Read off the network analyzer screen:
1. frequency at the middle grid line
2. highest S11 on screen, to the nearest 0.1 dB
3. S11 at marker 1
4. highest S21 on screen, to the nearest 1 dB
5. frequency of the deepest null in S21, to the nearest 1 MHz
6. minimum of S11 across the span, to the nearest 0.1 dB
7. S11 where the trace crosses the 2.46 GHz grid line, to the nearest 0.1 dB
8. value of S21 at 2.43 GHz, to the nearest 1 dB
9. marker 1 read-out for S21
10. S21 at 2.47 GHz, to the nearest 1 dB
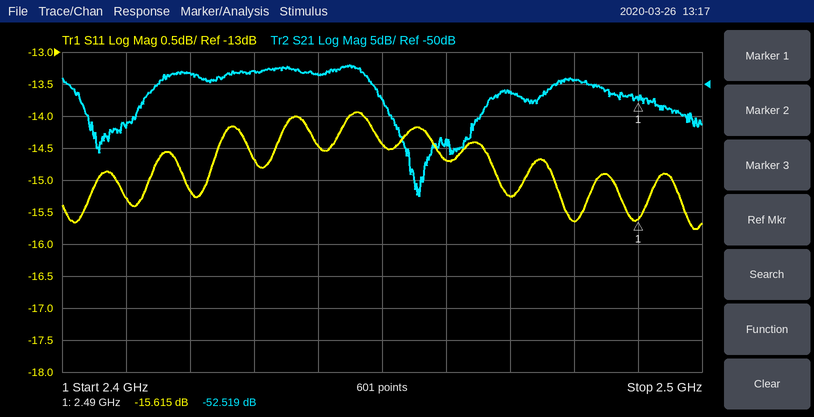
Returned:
2.45 GHz
-13.9 dB
-15.615 dB
-47 dB
2.456 GHz
-15.8 dB
-14.7 dB
-48 dB
-52.519 dB
-51 dB
